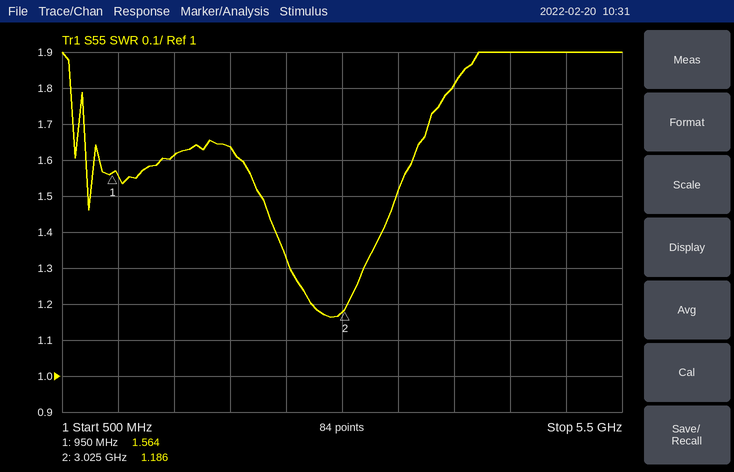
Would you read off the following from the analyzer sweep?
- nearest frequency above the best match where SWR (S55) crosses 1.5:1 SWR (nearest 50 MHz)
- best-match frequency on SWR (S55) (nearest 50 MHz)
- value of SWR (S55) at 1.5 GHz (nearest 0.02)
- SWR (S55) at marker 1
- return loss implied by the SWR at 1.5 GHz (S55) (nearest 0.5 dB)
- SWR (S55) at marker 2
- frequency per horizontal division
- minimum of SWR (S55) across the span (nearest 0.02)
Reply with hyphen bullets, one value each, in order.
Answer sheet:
- 3.50 GHz
- 2.90 GHz
- 1.62
- 1.564
- 12.5 dB
- 1.186
- 500 MHz
- 1.16
